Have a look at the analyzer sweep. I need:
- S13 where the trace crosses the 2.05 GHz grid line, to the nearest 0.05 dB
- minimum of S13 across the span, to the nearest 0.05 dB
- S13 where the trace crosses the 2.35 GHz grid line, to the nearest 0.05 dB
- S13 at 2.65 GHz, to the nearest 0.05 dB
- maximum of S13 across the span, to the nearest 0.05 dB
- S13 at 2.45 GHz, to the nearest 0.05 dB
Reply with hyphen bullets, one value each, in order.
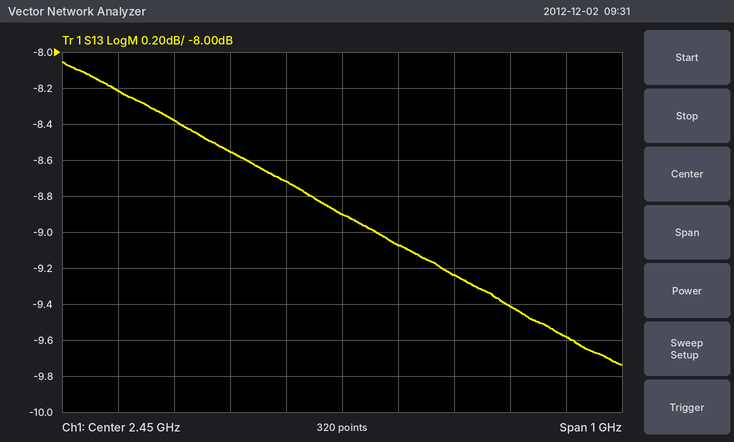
- -8.20 dB
- -9.75 dB
- -8.70 dB
- -9.25 dB
- -8.05 dB
- -8.90 dB
